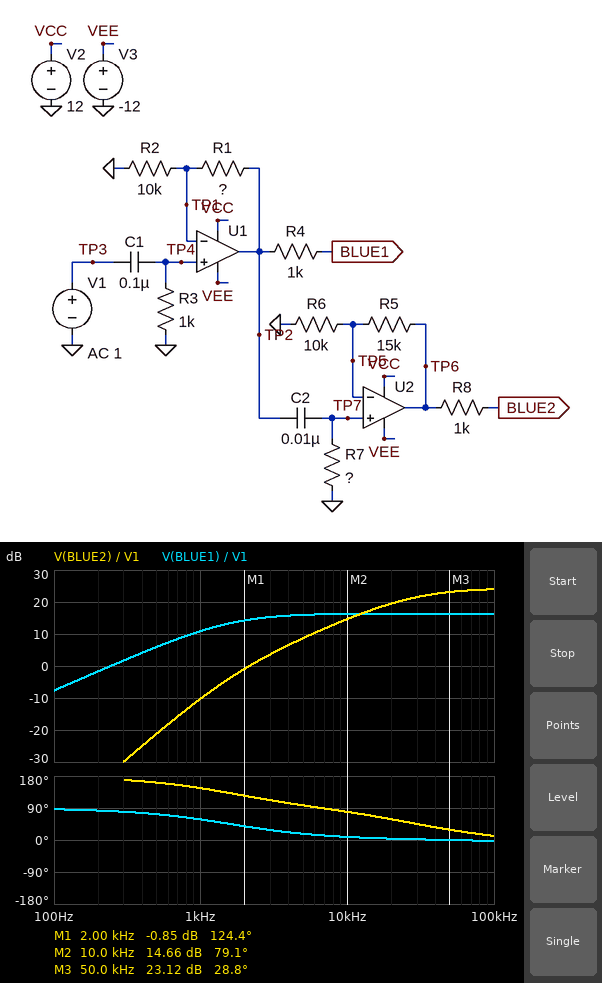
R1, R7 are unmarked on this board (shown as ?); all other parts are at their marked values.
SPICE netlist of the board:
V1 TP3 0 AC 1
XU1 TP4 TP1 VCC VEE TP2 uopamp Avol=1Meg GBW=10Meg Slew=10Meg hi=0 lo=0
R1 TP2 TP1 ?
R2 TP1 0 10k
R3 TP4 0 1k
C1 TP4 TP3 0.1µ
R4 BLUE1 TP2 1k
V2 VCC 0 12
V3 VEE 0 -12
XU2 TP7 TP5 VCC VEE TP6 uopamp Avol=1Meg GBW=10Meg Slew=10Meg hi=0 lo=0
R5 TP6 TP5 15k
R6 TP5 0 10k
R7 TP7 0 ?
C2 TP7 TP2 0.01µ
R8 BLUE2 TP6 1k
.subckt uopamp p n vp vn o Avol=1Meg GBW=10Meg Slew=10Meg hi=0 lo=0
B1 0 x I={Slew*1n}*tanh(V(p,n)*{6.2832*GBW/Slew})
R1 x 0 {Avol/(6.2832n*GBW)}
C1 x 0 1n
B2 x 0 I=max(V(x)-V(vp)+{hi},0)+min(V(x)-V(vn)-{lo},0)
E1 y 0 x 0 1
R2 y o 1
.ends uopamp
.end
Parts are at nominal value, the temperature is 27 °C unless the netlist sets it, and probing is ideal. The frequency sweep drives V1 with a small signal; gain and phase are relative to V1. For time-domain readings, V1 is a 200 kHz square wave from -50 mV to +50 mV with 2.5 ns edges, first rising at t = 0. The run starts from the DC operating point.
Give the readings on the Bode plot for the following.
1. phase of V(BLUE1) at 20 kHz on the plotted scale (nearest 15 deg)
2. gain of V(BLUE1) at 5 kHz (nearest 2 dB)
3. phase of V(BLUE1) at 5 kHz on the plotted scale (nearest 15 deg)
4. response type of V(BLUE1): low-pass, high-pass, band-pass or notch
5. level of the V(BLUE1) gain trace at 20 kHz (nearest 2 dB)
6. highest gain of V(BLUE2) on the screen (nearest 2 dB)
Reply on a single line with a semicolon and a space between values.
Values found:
0 deg; 16 dB; 15 deg; high-pass; 16 dB; 24 dB
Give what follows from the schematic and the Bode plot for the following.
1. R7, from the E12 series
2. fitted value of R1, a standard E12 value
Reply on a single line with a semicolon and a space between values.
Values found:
560 Ω; 56 kΩ
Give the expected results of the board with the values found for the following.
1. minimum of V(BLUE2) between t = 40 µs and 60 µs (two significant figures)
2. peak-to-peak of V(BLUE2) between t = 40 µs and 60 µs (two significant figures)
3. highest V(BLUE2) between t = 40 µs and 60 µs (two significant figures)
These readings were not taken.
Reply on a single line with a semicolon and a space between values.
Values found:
-960 mV; 1.9 V; 900 mV
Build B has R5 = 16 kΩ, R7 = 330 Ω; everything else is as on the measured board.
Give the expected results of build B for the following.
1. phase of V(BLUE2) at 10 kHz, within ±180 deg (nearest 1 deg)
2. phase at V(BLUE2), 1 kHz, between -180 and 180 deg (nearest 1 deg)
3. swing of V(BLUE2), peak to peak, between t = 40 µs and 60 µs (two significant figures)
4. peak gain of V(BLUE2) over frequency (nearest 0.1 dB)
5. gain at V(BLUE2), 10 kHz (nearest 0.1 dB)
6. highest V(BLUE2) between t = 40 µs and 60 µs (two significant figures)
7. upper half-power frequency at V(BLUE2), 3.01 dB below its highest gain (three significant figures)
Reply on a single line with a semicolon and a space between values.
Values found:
87 deg; 147 deg; 2.1 V; 24.4 dB; 10.7 dB; 1.0 V; 1.42 MHz
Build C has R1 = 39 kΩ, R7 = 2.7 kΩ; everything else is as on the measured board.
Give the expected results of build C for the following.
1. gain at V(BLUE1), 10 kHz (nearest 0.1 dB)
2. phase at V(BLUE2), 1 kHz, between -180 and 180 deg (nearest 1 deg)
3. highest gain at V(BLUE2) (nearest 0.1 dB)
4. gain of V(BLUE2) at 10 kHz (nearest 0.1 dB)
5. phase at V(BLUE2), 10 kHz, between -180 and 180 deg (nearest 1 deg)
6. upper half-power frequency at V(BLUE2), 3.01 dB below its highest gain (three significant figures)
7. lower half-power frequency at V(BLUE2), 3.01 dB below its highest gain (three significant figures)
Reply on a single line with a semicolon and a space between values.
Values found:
13.7 dB; 138 deg; 21.7 dB; 20.4 dB; 39 deg; 1.71 MHz; 6.25 kHz
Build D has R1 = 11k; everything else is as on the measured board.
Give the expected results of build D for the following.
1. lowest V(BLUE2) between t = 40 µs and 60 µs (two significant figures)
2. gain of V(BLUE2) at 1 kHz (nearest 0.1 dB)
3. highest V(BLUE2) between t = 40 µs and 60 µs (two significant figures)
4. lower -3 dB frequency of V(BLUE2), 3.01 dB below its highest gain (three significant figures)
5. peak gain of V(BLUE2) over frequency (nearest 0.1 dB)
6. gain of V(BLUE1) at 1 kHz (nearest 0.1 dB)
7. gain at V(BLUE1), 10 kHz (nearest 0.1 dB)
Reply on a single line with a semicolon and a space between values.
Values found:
-320 mV; -20.2 dB; 300 mV; 28.0 kHz; 14.3 dB; 1.0 dB; 6.3 dB
